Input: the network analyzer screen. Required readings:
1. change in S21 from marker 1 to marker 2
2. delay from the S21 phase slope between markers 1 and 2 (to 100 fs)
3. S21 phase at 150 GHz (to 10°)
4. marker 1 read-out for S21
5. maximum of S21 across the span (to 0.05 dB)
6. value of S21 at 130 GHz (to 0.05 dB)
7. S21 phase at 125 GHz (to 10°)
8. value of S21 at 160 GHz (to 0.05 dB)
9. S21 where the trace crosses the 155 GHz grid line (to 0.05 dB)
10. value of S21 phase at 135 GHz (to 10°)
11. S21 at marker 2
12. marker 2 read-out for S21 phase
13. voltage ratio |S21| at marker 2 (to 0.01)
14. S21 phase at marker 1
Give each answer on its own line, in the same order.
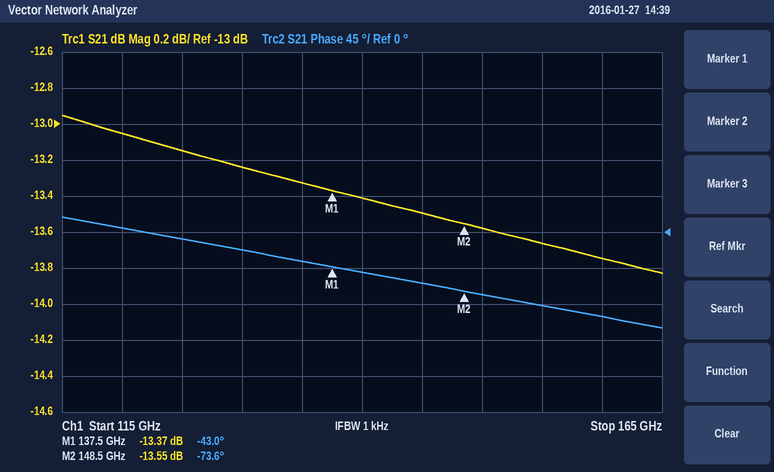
-0.18 dB
7.7 ps
-80°
-13.37 dB
-12.95 dB
-13.25 dB
-10°
-13.75 dB
-13.65 dB
-40°
-13.55 dB
-73.6°
0.21
-43.0°
